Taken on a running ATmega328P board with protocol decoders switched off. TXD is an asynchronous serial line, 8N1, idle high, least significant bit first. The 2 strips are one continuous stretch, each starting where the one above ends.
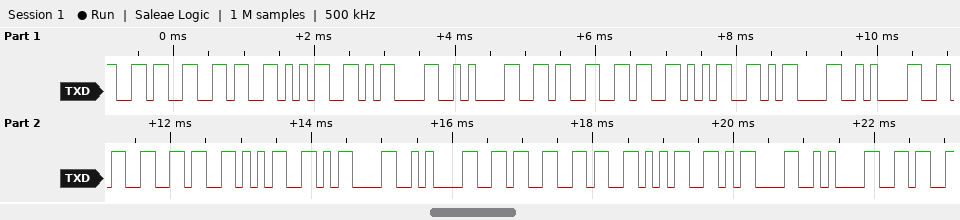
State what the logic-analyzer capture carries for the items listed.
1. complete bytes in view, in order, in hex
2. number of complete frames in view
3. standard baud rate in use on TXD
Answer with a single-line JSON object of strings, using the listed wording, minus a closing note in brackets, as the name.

{"complete bytes in view, in order, in hex": "0x36 0x36 0x35 0x0D 0x0A 0x36 0x36 0x35 0x0D 0x0A 0x36 0x36 0x35 0x0D 0x0A 0x36 0x36 0x35 0x0D 0x0A 0x36", "number of complete frames in view": "21", "standard baud rate in use on TXD": "9600 baud"}
